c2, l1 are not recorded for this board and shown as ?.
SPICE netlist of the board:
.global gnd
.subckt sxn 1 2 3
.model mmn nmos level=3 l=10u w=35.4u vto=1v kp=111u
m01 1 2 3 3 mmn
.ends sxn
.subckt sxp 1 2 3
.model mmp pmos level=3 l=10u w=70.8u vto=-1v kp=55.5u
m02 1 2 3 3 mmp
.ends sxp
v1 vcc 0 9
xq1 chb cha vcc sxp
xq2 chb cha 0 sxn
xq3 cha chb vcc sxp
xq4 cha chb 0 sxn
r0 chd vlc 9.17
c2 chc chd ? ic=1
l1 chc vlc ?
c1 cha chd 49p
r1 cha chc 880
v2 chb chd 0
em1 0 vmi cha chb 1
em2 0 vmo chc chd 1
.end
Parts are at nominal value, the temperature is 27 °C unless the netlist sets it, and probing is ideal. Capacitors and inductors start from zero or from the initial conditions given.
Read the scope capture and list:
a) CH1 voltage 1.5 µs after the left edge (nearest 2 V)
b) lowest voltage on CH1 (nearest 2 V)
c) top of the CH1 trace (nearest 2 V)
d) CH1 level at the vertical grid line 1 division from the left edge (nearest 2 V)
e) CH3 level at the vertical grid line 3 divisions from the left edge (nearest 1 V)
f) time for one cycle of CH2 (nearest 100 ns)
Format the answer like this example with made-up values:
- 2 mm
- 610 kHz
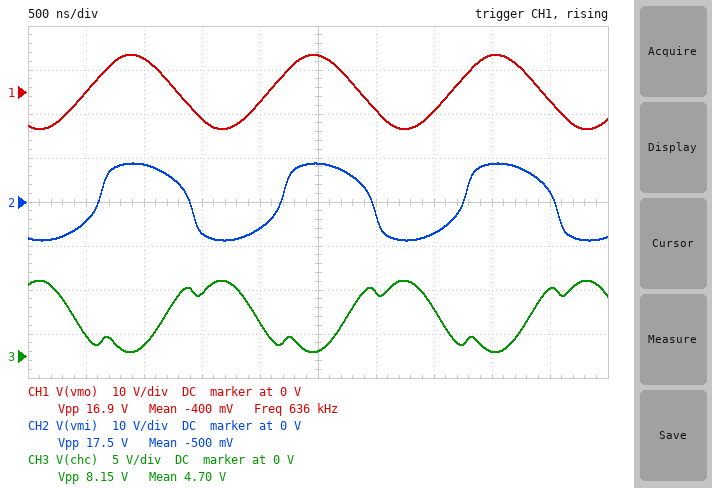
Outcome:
- -6 V
- -8 V
- 8 V
- 0 V
- 7 V
- 1.6 µs
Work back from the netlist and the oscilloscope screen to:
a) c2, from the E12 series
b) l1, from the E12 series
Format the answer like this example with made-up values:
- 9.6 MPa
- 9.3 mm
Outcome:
- 820 pF
- 68 µH
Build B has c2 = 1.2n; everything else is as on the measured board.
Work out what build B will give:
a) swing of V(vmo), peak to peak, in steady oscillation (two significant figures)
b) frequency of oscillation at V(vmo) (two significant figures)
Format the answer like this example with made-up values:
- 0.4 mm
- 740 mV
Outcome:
- 16 V
- 530 kHz
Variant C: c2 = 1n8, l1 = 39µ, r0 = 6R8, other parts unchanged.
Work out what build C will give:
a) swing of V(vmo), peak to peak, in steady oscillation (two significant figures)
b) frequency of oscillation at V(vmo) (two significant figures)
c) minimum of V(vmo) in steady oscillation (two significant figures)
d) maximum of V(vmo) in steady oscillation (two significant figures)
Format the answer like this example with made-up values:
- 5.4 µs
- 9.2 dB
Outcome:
- 13 V
- 580 kHz
- -6.4 V
- 6.4 V
